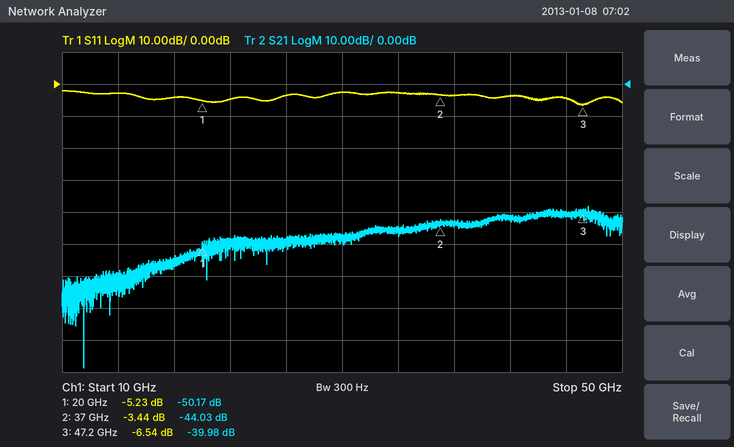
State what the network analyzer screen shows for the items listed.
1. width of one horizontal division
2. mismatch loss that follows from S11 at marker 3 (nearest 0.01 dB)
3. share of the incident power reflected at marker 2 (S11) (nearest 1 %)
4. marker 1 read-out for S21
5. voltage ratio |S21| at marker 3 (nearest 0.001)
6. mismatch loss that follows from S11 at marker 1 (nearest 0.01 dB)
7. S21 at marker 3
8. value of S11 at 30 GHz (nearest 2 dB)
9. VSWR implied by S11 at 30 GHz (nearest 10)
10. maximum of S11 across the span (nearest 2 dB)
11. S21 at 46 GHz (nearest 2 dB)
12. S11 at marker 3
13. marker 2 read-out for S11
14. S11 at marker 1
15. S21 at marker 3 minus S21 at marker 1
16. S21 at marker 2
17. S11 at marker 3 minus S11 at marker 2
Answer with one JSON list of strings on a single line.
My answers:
["4 GHz", "1.09 dB", "45 %", "-50.17 dB", "0.010", "1.55 dB", "-39.98 dB", "-2 dB", "10", "-2 dB", "-40 dB", "-6.54 dB", "-3.44 dB", "-5.23 dB", "10.19 dB", "-44.03 dB", "-3.10 dB"]
